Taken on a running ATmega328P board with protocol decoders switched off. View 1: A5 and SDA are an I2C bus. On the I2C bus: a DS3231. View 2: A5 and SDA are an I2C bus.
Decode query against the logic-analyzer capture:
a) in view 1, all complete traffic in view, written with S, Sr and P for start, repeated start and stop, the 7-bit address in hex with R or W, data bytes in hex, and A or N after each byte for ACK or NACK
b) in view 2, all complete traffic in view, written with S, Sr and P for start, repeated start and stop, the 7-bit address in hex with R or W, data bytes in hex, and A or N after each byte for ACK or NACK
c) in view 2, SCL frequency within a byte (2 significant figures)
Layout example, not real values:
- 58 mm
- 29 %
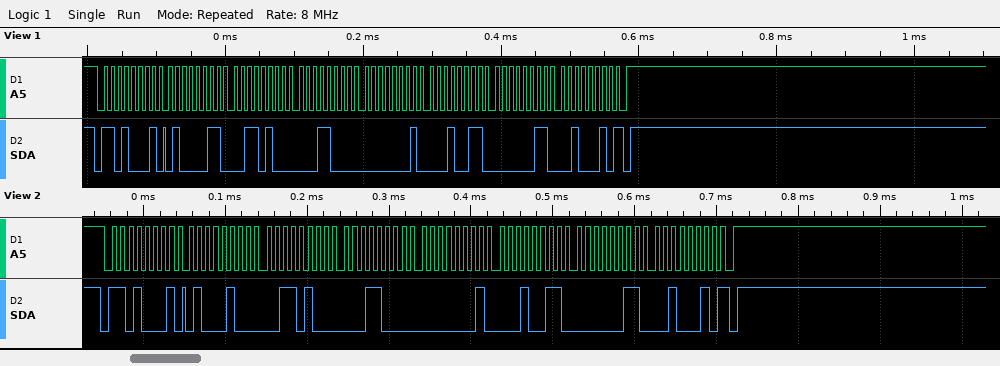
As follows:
- S 68R A 43 A 34 A 18 A 01 A 13 A 03 A 22 N P
- S 68R A 44 A 34 A 18 A 01 A 13 A 03 A 22 N P
- 100 kHz
